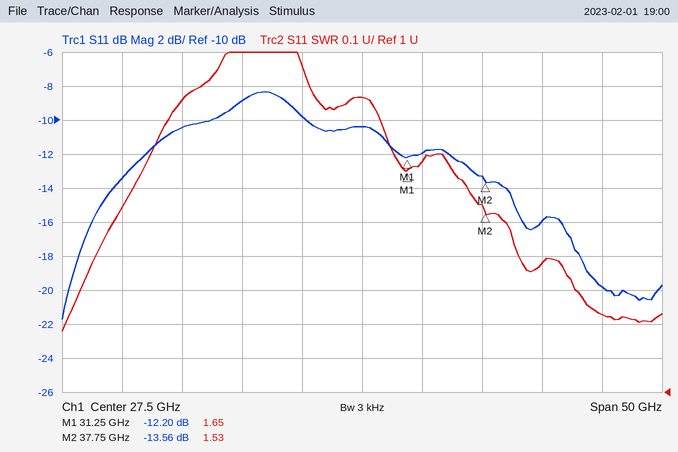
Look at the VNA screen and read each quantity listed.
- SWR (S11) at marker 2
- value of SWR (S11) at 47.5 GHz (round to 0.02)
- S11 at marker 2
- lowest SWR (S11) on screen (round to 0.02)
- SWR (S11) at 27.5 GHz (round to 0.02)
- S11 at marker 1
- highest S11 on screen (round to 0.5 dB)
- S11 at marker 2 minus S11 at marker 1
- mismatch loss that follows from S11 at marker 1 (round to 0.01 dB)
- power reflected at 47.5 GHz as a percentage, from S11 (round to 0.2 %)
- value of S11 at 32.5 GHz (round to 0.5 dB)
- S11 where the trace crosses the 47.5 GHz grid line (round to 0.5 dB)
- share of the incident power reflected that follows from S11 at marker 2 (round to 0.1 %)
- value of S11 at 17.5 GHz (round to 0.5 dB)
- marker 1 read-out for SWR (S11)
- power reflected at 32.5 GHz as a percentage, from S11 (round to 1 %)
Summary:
1.53
1.22
-13.56 dB
1.18
1.86
-12.20 dB
-8.5 dB
-1.36 dB
0.27 dB
1.0 %
-12.0 dB
-20.0 dB
4.4 %
-9.0 dB
1.65
6 %
